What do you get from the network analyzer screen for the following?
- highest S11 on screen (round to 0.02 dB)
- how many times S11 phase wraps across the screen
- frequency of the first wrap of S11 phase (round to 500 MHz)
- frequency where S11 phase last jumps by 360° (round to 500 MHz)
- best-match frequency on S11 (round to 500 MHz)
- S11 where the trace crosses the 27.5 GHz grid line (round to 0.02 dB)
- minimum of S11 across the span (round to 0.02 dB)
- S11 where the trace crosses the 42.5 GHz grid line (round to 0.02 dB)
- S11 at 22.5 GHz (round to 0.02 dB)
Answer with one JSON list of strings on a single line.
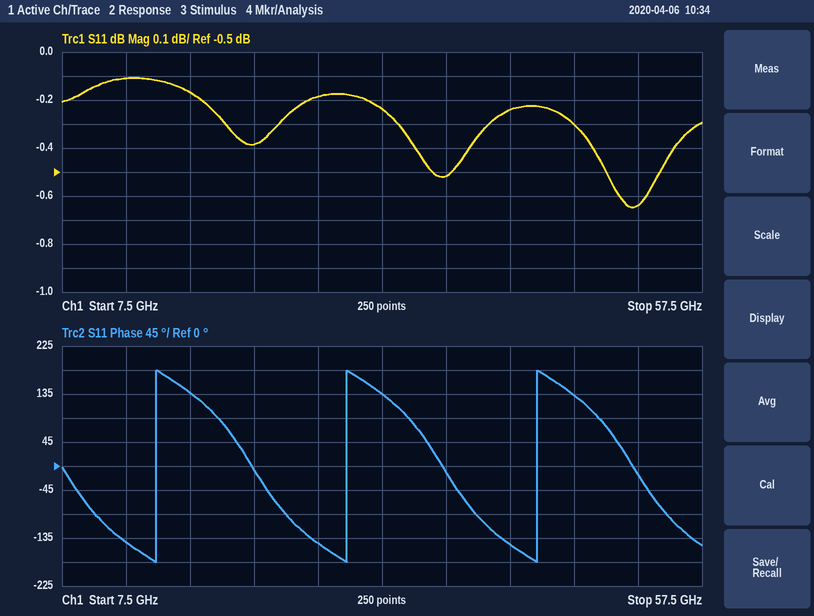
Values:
["-0.10 dB", "3", "15.0 GHz", "44.5 GHz", "52.0 GHz", "-0.18 dB", "-0.64 dB", "-0.24 dB", "-0.38 dB"]
